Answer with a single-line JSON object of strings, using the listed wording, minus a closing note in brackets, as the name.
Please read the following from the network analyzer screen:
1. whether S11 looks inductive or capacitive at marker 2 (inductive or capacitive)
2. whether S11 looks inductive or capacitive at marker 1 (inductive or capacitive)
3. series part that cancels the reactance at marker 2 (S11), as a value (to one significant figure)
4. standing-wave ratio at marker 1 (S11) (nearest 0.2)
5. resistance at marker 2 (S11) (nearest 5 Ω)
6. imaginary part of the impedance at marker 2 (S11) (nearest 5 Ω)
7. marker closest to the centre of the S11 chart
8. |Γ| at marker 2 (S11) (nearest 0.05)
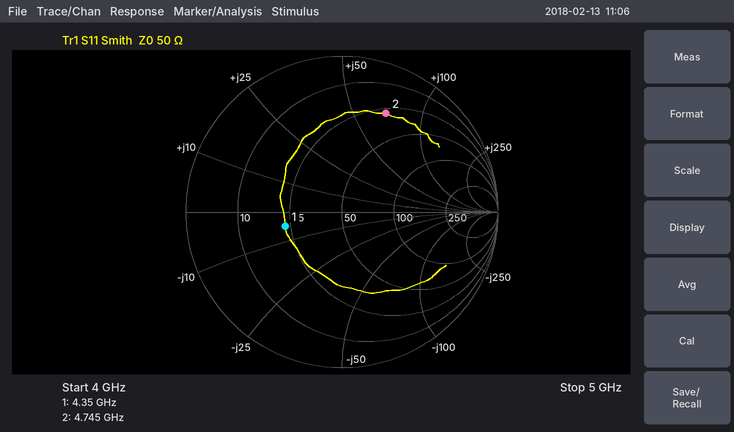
{"whether S11 looks inductive or capacitive at marker 2": "inductive", "whether S11 looks inductive or capacitive at marker 1": "capacitive", "series part that cancels the reactance at marker 2 (S11), as a value": "500 fF", "standing-wave ratio at marker 1 (S11)": "2.2", "resistance at marker 2 (S11)": "30 Ω", "imaginary part of the impedance at marker 2 (S11)": "+70 Ω", "marker closest to the centre of the S11 chart": "marker 1", "|Γ| at marker 2 (S11)": "0.70"}
